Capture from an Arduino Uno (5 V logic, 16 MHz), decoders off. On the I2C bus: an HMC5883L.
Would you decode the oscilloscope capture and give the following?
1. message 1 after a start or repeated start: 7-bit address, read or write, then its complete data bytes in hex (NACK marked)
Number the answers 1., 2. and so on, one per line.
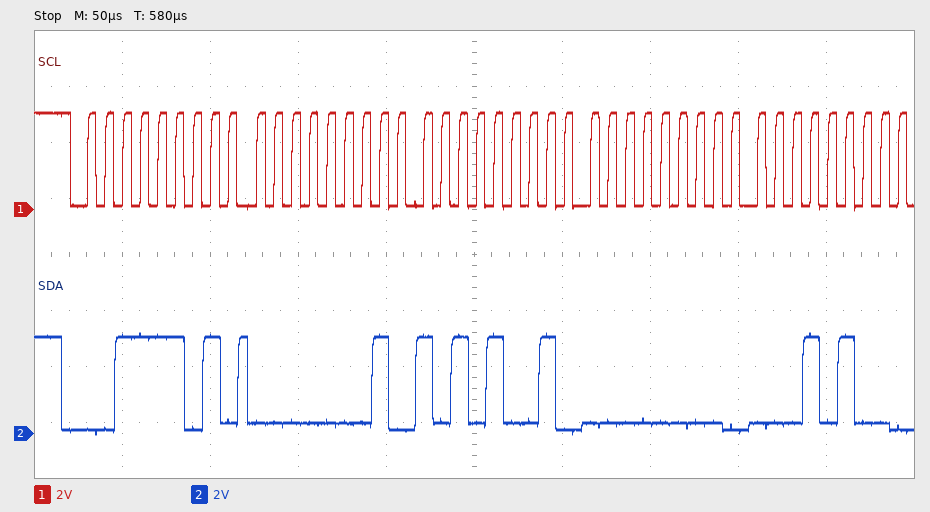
1. 0x1E read: 01 A9 00 14
